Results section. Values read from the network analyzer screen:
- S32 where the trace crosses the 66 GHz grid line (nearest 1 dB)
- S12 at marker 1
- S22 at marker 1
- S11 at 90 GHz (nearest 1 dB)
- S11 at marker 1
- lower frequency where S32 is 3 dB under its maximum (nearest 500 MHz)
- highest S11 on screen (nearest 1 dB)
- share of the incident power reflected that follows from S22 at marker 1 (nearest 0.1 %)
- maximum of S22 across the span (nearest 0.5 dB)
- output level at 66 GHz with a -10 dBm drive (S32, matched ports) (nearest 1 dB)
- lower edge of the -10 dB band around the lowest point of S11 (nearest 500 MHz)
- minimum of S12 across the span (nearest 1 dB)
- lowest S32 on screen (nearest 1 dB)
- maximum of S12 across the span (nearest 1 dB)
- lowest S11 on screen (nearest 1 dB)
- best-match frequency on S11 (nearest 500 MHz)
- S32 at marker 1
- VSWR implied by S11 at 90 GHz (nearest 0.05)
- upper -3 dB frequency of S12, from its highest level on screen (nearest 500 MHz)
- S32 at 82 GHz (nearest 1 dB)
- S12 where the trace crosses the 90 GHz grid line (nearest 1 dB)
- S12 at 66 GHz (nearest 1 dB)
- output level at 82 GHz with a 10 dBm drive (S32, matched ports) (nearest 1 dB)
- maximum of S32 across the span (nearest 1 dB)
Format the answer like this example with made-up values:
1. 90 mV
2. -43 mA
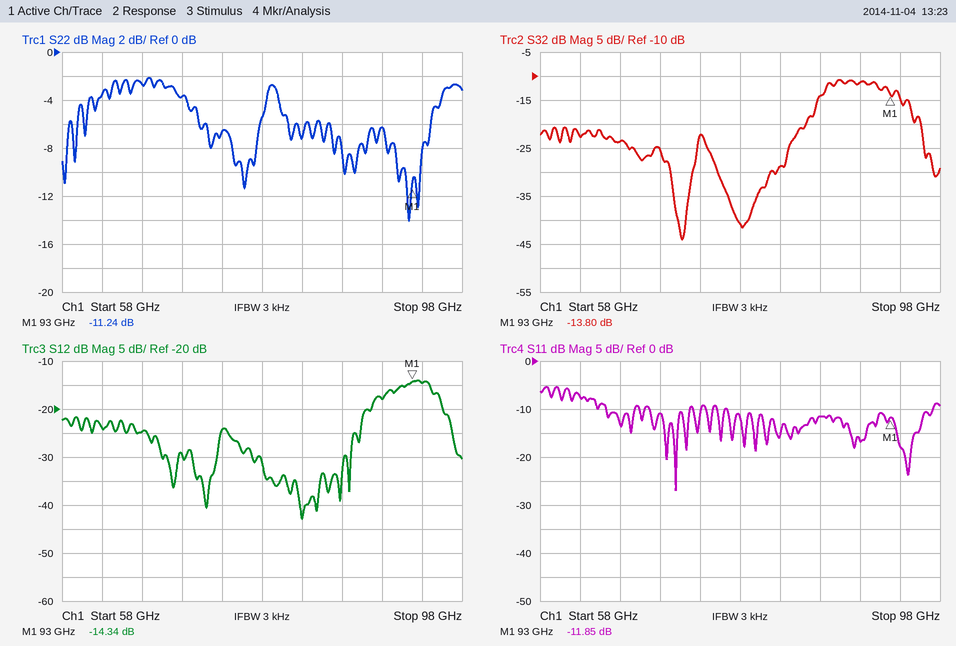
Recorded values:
1. -24 dB
2. -14.34 dB
3. -11.24 dB
4. -17 dB
5. -11.85 dB
6. 86.5 GHz
7. -5 dB
8. 7.5 %
9. -2.0 dB
10. -34 dBm
11. 69.0 GHz
12. -43 dB
13. -44 dB
14. -14 dB
15. -27 dB
16. 71.5 GHz
17. -13.80 dB
18. 1.35
19. 95.5 GHz
20. -29 dB
21. -18 dB
22. -25 dB
23. -19 dBm
24. -11 dB
